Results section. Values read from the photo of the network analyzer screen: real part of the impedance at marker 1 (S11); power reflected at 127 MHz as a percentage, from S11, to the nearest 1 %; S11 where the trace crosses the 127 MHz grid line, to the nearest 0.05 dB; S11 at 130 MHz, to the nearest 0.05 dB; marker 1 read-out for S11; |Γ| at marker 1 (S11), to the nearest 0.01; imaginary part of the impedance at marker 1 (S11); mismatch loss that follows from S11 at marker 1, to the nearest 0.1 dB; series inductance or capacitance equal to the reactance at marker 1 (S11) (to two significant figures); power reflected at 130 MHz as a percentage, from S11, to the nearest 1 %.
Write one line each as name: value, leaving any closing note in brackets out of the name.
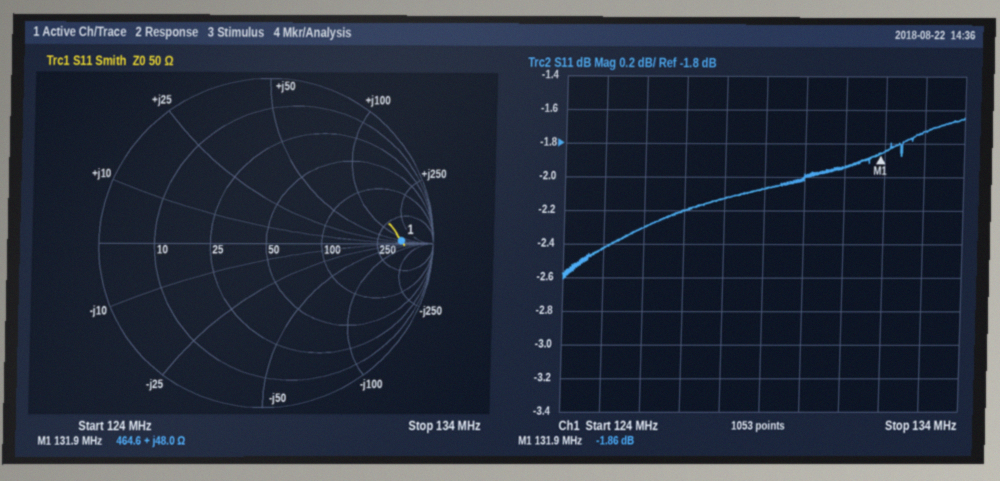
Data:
real part of the impedance at marker 1: 464.6 Ω
power reflected at 127 MHz as a percentage, from S11, to the nearest 1 %: 60 %
S11 where the trace crosses the 127 MHz grid line, to the nearest 0.05 dB: -2.20 dB
S11 at 130 MHz, to the nearest 0.05 dB: -2.00 dB
marker 1 read-out for S11: -1.86 dB
|Γ| at marker 1 (S11), to the nearest 0.01: 0.81
imaginary part of the impedance at marker 1: +48.0 Ω
mismatch loss that follows from S11 at marker 1, to the nearest 0.1 dB: 4.6 dB
series inductance or capacitance equal to the reactance at marker 1 (S11): 58 nH
power reflected at 130 MHz as a percentage, from S11, to the nearest 1 %: 63 %
